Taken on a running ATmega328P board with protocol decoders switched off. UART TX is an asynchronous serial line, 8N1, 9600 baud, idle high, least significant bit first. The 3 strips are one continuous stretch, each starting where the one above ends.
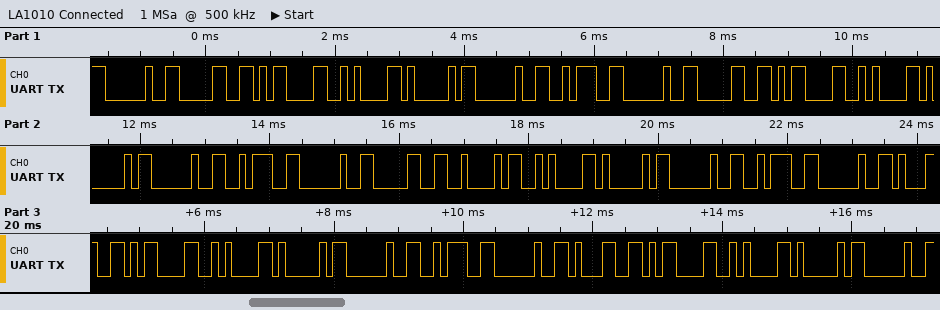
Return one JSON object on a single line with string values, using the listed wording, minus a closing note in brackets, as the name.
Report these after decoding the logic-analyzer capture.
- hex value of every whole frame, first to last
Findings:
{"hex value of every whole frame, first to last": "0x20 0x30 0x0D 0x0A 0x41 0x20 0x3A 0x20 0x30 0x0D 0x0A 0x41 0x20 0x3A 0x20 0x30 0x42 0x0A 0x41 0x20 0x3A 0x20 0x31 0x0D 0x0A 0x41 0x20 0x3A 0x20 0x31 0x0D 0x0A 0x41 0x20"}
